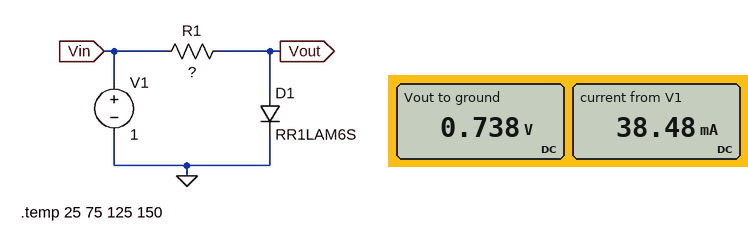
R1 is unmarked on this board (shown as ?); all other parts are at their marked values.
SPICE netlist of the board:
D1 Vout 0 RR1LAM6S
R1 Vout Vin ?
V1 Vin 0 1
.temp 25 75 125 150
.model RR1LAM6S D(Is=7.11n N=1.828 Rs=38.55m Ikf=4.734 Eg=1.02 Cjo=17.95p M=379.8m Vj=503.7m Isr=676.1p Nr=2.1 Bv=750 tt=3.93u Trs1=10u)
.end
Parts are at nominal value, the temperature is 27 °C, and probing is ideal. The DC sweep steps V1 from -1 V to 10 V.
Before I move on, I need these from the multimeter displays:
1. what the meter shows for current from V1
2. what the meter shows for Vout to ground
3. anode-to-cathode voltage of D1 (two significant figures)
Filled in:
38.48 mA
0.738 V
740 mV
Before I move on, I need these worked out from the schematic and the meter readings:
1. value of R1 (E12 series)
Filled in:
6.8 Ω
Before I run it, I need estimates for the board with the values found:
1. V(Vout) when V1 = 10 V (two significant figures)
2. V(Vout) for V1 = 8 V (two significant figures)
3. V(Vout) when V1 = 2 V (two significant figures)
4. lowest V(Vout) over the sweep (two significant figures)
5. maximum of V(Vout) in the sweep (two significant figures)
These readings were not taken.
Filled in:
980 mV
950 mV
820 mV
-1.0 V
980 mV
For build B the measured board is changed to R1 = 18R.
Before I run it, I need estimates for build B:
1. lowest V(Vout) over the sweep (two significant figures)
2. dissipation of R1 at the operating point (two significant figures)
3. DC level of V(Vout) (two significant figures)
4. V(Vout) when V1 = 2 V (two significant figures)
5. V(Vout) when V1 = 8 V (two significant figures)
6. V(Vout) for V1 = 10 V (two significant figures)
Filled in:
-1.0 V
5.1 mW
700 mV
770 mV
870 mV
890 mV
